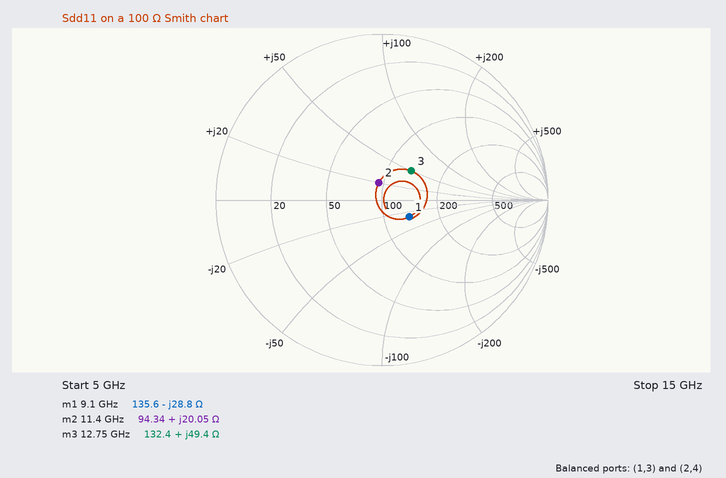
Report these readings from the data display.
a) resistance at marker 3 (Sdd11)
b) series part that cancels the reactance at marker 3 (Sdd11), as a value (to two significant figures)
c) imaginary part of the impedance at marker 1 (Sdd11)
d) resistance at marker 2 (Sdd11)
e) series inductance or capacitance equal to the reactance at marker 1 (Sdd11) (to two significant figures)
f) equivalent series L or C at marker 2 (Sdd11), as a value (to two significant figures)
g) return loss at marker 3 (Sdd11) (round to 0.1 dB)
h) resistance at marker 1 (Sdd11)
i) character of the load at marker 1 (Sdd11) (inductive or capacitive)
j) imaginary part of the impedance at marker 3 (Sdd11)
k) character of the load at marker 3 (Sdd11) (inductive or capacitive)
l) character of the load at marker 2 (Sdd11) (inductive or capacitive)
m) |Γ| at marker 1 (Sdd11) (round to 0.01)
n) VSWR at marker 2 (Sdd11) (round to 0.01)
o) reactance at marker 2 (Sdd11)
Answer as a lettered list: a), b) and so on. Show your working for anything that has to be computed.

a) 132.4 Ω
b) C = 1/(2π × 12.75 GHz × 49.4 Ω) ≈ 253 fF, so 250 fF to two significant figures
c) -28.8 Ω
d) 94.34 Ω
e) C = 1/(2π × 9.1 GHz × 28.8 Ω) ≈ 607 fF, so 610 fF to two significant figures
f) L = 20.05 Ω/(2π × 11.4 GHz) ≈ 280 pH
g) 12.1 dB
h) 135.6 Ω
i) capacitive
j) +49.4 Ω
k) inductive
l) inductive
m) 0.19
n) 1.24
o) +20.05 Ω
